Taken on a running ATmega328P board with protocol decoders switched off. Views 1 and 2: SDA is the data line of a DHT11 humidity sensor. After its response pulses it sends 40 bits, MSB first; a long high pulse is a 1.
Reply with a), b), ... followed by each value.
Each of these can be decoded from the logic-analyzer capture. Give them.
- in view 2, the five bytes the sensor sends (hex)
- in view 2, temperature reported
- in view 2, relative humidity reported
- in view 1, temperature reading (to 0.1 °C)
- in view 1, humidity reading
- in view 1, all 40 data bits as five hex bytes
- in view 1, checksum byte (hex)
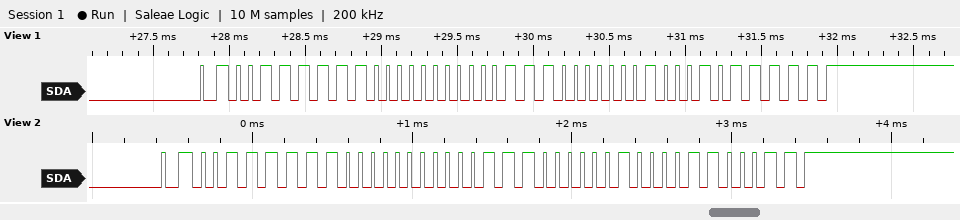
a) 3F 00 1C 08 63
b) 28.8 °C
c) 63 %
d) 28.4 °C
e) 63 %
f) 3F 00 1C 04 5F
g) 0x5F
